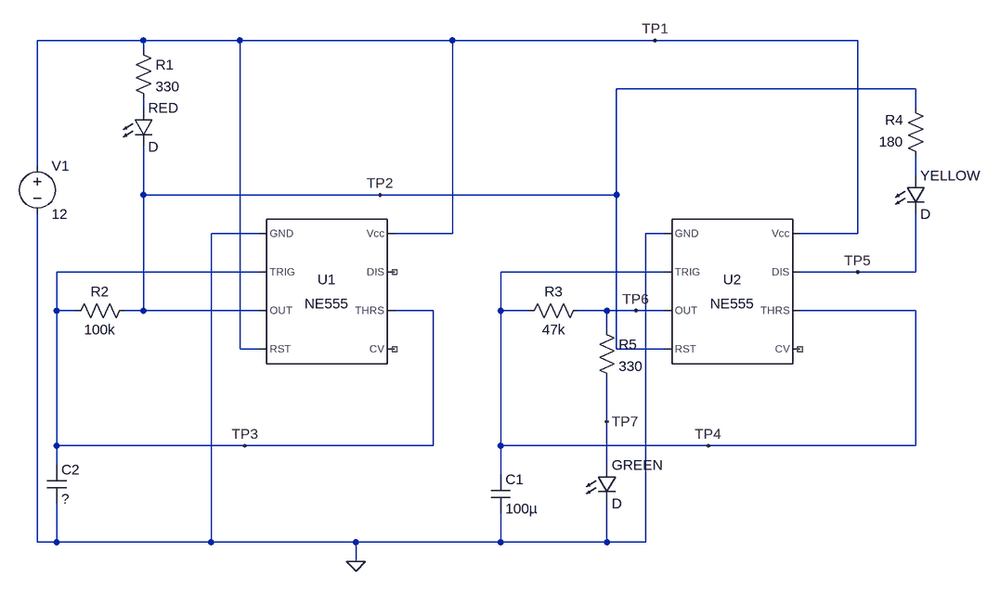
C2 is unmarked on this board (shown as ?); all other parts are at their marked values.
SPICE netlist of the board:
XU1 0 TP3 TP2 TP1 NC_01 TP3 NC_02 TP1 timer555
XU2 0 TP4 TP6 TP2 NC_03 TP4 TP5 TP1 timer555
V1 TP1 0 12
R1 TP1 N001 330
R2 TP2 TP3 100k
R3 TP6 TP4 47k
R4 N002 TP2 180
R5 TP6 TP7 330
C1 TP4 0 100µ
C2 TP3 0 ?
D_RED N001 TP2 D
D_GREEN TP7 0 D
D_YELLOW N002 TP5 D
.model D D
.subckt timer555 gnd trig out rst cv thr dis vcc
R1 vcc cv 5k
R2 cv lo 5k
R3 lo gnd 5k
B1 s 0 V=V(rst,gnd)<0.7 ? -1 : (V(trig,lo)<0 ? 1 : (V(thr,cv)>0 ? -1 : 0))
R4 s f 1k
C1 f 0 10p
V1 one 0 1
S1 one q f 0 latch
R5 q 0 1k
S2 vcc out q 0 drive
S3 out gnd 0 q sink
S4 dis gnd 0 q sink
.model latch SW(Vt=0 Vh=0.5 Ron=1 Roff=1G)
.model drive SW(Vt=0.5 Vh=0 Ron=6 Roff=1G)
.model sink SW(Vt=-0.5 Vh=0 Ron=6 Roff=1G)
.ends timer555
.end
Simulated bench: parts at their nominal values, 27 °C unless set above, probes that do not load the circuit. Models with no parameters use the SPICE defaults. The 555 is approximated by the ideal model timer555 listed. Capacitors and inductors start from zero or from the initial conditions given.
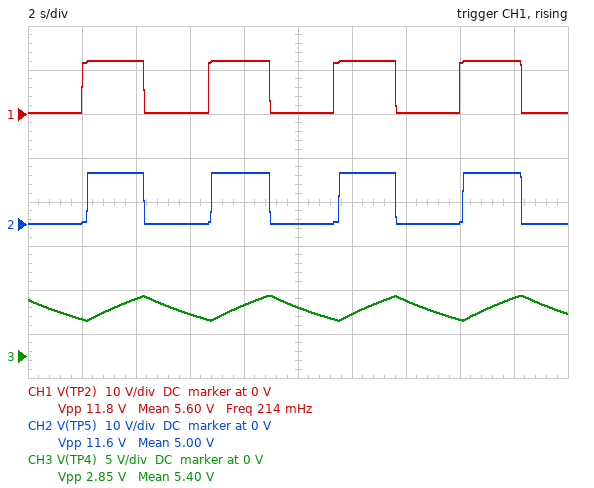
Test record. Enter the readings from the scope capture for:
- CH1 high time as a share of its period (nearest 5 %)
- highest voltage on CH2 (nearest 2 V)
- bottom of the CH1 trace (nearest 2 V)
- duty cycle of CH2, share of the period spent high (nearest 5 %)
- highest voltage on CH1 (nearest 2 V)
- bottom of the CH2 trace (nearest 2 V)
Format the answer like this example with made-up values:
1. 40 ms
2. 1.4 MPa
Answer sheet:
1. 50 %
2. 12 V
3. 0 V
4. 45 %
5. 12 V
6. 0 V
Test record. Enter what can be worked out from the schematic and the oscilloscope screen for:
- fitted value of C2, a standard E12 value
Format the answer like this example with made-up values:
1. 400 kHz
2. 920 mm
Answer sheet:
1. 33 µF
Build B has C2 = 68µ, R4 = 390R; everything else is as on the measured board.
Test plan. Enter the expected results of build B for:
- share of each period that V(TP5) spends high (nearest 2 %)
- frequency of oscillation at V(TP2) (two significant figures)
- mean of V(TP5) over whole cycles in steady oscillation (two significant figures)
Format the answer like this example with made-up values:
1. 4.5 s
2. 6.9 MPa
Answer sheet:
1. 44 %
2. 100 mHz
3. 5.1 V
